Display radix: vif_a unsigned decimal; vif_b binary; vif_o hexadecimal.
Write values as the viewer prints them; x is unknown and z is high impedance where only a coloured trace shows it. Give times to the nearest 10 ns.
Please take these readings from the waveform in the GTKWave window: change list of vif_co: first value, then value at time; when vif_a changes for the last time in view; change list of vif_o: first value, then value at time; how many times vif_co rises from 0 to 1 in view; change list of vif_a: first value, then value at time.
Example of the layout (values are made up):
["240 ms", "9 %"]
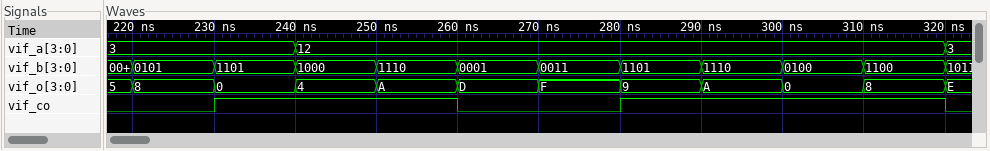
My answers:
["0, 1 at 230 ns, 0 at 260 ns, 1 at 280 ns, 0 at 320 ns", "320 ns", "5, 8 at 220 ns, 0 at 230 ns, 4 at 240 ns, A at 250 ns, D at 260 ns, F at 270 ns, 9 at 280 ns, A at 290 ns, 0 at 300 ns, 8 at 310 ns, E at 320 ns", "2", "3, 12 at 240 ns, 3 at 320 ns"]
